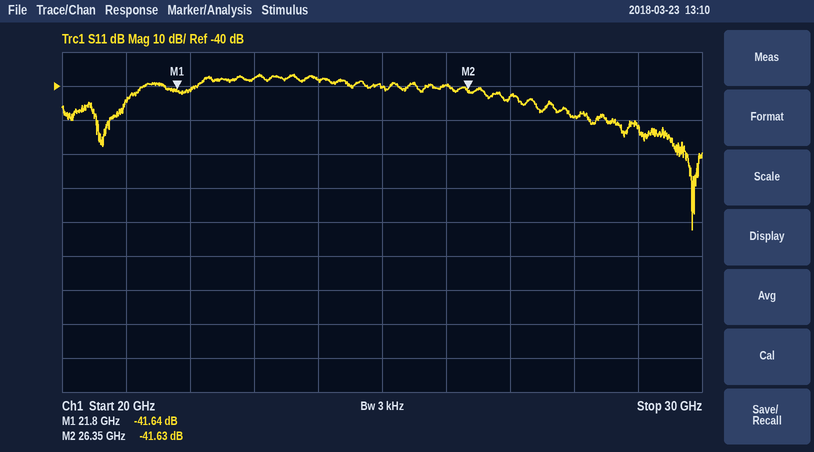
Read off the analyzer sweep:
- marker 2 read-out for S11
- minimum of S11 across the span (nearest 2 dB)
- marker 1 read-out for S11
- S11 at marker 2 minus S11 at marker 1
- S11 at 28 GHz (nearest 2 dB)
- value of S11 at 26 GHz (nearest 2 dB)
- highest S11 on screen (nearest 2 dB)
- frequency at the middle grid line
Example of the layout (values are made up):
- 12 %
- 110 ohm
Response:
- -41.63 dB
- -82 dB
- -41.64 dB
- 0.01 dB
- -50 dB
- -40 dB
- -36 dB
- 25 GHz
